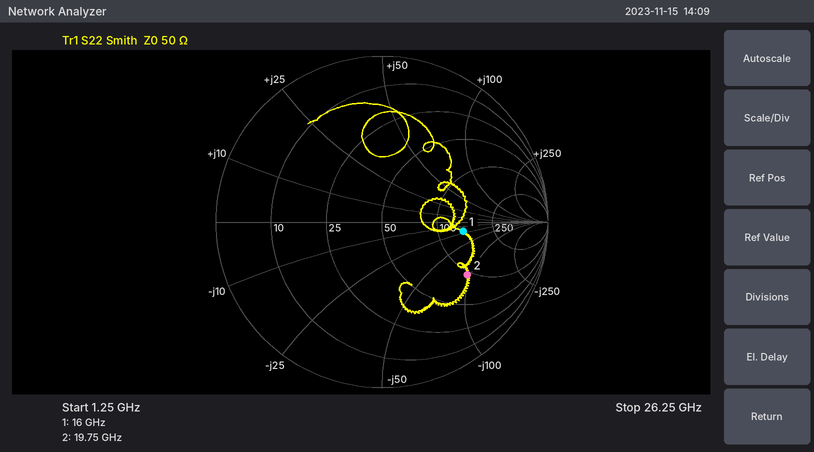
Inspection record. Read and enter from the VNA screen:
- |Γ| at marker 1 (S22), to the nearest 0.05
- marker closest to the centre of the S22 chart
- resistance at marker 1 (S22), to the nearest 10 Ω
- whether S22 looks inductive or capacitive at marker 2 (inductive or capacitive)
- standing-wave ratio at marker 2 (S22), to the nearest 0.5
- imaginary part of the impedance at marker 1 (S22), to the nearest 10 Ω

0.50
marker 1
140 Ω
capacitive
4.0
-20 Ω
